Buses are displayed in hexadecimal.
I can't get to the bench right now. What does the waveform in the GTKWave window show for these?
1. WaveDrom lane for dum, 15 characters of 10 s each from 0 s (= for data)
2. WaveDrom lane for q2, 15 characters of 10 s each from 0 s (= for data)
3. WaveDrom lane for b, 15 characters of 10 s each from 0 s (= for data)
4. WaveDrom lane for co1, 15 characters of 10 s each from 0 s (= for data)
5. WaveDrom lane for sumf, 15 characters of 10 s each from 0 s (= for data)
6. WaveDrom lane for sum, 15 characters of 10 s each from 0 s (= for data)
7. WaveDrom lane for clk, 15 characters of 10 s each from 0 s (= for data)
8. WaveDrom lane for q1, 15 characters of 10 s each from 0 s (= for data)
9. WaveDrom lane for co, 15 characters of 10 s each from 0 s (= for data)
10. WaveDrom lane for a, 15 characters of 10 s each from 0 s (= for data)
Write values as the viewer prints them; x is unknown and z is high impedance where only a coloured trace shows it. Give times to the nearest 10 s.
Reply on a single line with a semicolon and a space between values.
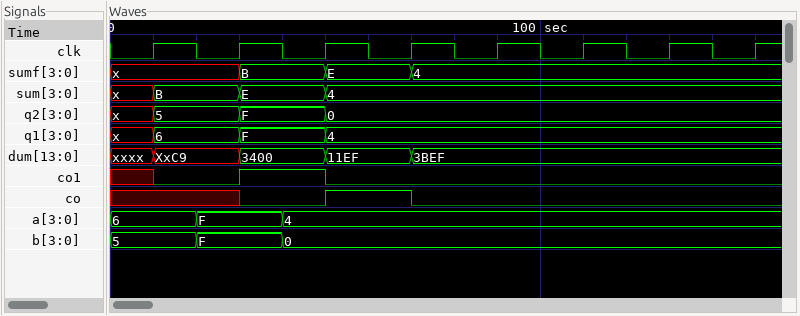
{name: 'dum', wave: 'x=.=.=.=.......', data: 'XxC9 3400 11EF 3BEF'}; {name: 'q2', wave: 'x=.=.=.........', data: '5 F 0'}; {name: 'b', wave: '=.=.=..........', data: '5 F 0'}; {name: 'co1', wave: 'x0.1.0.........'}; {name: 'sumf', wave: 'x..=.=.=.......', data: 'B E 4'}; {name: 'sum', wave: 'x=.=.=.........', data: 'B E 4'}; {name: 'clk', wave: '010101010101010'}; {name: 'q1', wave: 'x=.=.=.........', data: '6 F 4'}; {name: 'co', wave: 'x..0.1.0.......'}; {name: 'a', wave: '=.=.=..........', data: '6 F 4'}
